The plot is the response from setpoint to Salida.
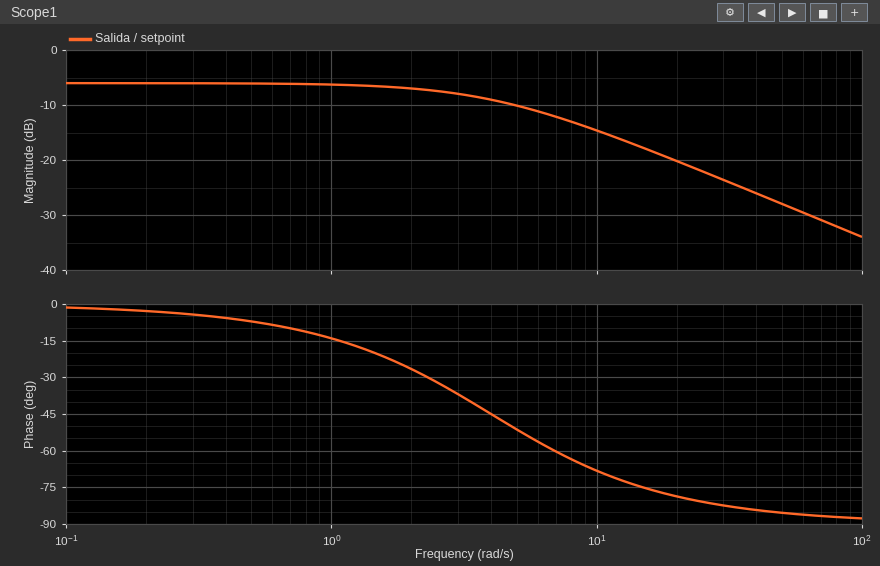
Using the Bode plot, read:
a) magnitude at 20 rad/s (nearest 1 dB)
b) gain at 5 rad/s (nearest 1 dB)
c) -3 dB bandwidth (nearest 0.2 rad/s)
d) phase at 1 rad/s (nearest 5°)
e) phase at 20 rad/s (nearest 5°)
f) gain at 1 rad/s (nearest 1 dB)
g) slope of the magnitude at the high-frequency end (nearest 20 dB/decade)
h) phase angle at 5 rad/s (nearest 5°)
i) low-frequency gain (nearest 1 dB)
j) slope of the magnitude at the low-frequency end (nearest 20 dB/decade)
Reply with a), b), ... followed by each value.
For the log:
a) -20 dB
b) -10 dB
c) 4.0 rad/s
d) -15°
e) -80°
f) -6 dB
g) -20 dB/decade
h) -50°
i) -6 dB
j) 0 dB/decade
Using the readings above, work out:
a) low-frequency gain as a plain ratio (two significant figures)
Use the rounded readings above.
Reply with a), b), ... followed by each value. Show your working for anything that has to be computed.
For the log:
a) 10^(-6 / 20) = 0.50
